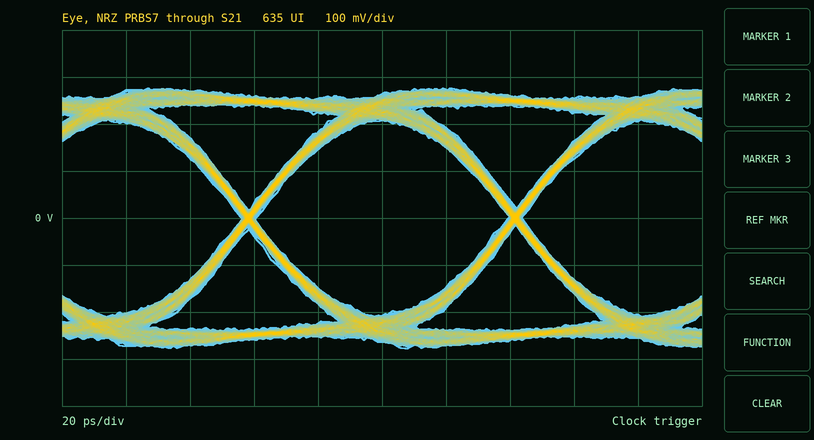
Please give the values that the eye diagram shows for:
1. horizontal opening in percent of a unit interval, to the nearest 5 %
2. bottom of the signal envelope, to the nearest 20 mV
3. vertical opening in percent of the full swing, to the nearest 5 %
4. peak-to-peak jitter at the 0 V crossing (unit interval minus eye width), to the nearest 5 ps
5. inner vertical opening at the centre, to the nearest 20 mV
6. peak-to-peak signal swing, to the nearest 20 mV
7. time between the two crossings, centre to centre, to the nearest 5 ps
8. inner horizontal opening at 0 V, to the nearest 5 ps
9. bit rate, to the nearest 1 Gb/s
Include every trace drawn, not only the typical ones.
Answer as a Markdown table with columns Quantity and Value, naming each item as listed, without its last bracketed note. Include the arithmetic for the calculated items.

| Quantity | Value |
|---|---|
| horizontal opening in percent of a unit interval, to the nearest 5 % | 80 ps / 85 ps ≈ 94.1 %, so 95 % to the nearest 5 % |
| bottom of the signal envelope, to the nearest 20 mV | -280 mV |
| vertical opening in percent of the full swing, to the nearest 5 % | 420 mV / 560 mV ≈ 75 % |
| peak-to-peak jitter at the 0 V crossing (unit interval minus eye width), to the nearest 5 ps | 5 ps |
| inner vertical opening at the centre, to the nearest 20 mV | 420 mV |
| peak-to-peak signal swing, to the nearest 20 mV | 560 mV |
| time between the two crossings, centre to centre, to the nearest 5 ps | 85 ps |
| inner horizontal opening at 0 V, to the nearest 5 ps | 80 ps |
| bit rate, to the nearest 1 Gb/s | 12 Gb/s |
